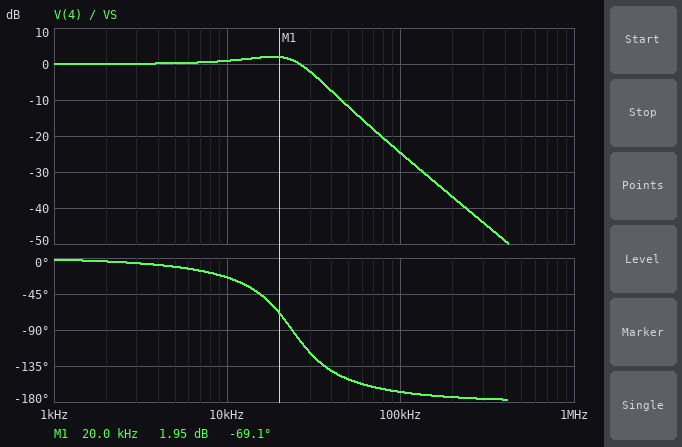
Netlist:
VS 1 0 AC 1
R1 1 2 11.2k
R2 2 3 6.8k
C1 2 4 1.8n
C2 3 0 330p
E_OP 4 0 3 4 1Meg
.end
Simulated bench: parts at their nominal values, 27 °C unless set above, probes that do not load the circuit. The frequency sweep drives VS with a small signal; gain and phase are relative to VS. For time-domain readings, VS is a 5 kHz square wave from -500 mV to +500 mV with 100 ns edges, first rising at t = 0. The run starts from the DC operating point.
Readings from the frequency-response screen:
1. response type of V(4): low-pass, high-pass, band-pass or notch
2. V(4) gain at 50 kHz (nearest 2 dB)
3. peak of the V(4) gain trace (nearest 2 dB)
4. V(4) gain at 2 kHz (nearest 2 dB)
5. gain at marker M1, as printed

low-pass
-12 dB
2 dB
0 dB
1.95 dB
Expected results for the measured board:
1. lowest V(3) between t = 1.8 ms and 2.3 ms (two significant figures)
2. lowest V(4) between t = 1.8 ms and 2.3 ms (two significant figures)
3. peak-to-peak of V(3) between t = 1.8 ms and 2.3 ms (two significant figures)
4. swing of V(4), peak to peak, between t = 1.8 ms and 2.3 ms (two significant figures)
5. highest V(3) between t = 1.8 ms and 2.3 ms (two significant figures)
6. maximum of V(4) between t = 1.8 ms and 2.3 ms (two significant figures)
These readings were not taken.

-710 mV
-710 mV
1.4 V
1.4 V
710 mV
710 mV
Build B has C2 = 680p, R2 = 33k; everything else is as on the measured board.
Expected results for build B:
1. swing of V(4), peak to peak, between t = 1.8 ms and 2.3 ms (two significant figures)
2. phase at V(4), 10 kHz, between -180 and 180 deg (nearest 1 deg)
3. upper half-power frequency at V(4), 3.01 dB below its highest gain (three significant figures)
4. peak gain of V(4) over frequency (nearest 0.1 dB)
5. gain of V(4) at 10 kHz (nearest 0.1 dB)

1.1 V
-113 deg
7.49 kHz
0 dB
-6.2 dB
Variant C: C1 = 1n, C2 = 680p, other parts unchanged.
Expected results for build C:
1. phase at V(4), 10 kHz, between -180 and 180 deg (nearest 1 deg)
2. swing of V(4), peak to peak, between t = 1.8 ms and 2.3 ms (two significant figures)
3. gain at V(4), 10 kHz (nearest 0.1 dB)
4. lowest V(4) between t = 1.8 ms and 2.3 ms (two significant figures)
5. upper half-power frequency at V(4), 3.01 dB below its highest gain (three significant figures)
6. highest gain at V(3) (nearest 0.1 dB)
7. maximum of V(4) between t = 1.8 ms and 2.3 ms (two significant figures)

-44 deg
1.0 V
-0.9 dB
-510 mV
17.8 kHz
0 dB
510 mV
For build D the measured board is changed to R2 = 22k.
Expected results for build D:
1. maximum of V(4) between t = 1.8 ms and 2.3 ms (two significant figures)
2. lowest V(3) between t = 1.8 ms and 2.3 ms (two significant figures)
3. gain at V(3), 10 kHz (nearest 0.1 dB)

700 mV
-700 mV
1.9 dB
